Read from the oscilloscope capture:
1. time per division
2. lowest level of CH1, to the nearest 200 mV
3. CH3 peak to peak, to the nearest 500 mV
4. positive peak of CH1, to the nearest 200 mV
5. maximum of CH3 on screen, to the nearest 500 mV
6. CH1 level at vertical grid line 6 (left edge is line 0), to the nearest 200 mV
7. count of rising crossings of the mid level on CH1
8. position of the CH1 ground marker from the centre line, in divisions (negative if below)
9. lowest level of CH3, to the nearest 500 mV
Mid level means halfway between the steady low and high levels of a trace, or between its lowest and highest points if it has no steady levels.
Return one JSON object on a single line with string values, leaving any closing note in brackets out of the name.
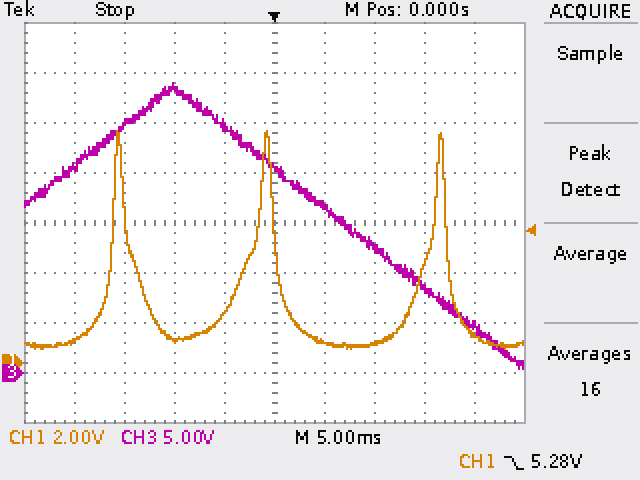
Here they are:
{"time per division": "5 ms", "lowest level of CH1, to the nearest 200 mV": "600 mV", "CH3 peak to peak, to the nearest 500 mV": "28.5 V", "positive peak of CH1, to the nearest 200 mV": "9.2 V", "maximum of CH3 on screen, to the nearest 500 mV": "29.0 V", "CH1 level at vertical grid line 6 (left edge is line 0), to the nearest 200 mV": "800 mV", "count of rising crossings of the mid level on CH1": "3", "position of the CH1 ground marker from the centre line, in divisions": "-2.8 div", "lowest level of CH3, to the nearest 500 mV": "500 mV"}
